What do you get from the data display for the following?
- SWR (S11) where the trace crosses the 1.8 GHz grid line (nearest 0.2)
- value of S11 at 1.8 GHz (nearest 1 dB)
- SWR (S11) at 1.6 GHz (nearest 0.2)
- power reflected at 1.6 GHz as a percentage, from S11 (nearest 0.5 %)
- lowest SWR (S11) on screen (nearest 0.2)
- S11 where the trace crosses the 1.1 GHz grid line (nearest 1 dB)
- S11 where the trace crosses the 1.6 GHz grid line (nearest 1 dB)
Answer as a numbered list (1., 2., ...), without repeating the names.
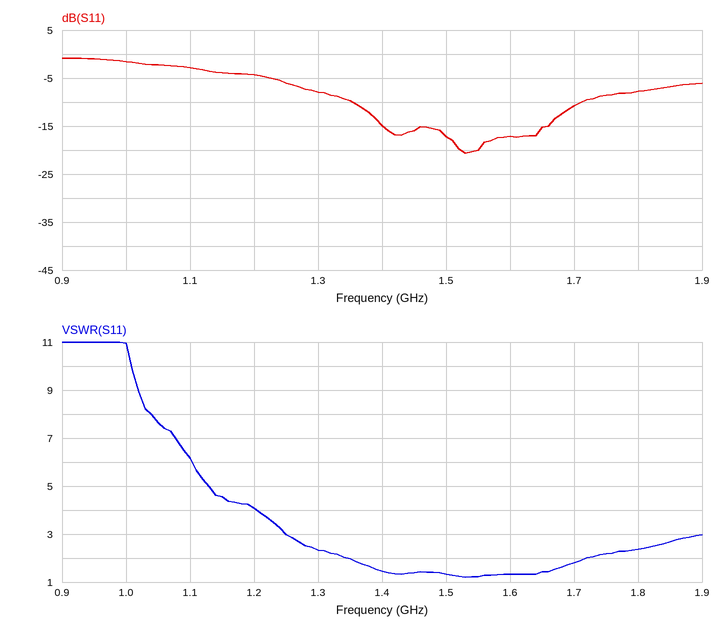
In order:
1. 2.4
2. -8 dB
3. 1.4
4. 2.0 %
5. 1.2
6. -3 dB
7. -17 dB
